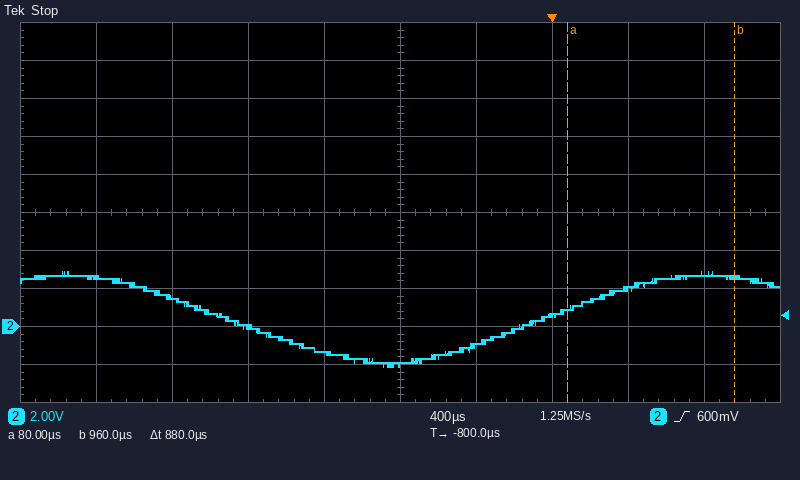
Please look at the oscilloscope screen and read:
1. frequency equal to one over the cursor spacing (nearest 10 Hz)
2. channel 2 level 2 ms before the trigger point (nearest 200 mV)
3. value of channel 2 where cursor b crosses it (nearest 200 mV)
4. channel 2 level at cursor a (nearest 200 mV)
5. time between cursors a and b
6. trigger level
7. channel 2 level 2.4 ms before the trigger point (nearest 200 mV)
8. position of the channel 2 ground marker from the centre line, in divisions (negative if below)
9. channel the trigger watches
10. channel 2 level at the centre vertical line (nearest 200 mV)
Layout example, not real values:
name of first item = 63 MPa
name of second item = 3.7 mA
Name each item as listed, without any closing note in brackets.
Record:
frequency equal to one over the cursor spacing = 1.14 kHz
channel 2 level 2 ms before the trigger point = 1.6 V
value of channel 2 where cursor b crosses it = 2.6 V
channel 2 level at cursor a = 1.0 V
time between cursors a and b = 880 µs
trigger level = 600 mV
channel 2 level 2.4 ms before the trigger point = 2.6 V
position of the channel 2 ground marker from the centre line, in divisions = -3.0 div
channel the trigger watches = channel 2
channel 2 level at the centre vertical line = -2.0 V
